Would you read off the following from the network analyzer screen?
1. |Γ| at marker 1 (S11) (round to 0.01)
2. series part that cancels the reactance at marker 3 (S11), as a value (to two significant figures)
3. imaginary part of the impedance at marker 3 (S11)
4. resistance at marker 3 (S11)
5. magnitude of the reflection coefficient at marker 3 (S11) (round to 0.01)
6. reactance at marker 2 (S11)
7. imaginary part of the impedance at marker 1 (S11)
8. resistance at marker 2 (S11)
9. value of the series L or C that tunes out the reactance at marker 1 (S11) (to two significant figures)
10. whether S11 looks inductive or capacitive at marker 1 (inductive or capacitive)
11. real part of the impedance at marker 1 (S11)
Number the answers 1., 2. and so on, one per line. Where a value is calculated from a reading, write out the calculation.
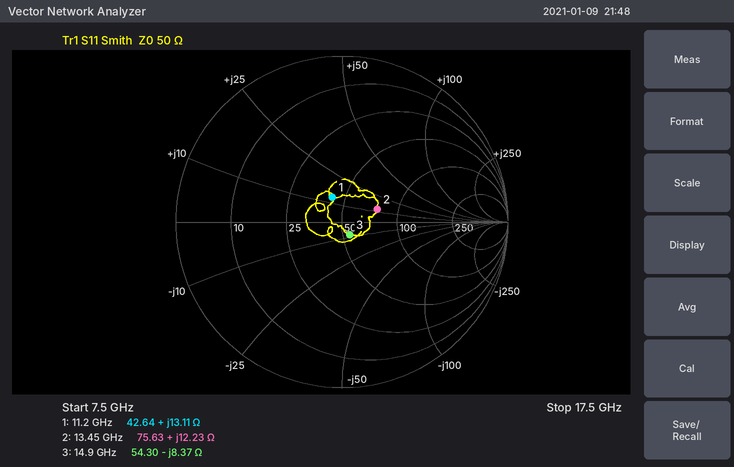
1. 0.16
2. L = 8.37 Ω/(2π × 14.9 GHz) ≈ 89 pH
3. -8.37 Ω
4. 54.30 Ω
5. 0.09
6. +12.23 Ω
7. +13.11 Ω
8. 75.63 Ω
9. C = 1/(2π × 11.2 GHz × 13.11 Ω) ≈ 1.1 pF
10. inductive
11. 42.64 Ω
